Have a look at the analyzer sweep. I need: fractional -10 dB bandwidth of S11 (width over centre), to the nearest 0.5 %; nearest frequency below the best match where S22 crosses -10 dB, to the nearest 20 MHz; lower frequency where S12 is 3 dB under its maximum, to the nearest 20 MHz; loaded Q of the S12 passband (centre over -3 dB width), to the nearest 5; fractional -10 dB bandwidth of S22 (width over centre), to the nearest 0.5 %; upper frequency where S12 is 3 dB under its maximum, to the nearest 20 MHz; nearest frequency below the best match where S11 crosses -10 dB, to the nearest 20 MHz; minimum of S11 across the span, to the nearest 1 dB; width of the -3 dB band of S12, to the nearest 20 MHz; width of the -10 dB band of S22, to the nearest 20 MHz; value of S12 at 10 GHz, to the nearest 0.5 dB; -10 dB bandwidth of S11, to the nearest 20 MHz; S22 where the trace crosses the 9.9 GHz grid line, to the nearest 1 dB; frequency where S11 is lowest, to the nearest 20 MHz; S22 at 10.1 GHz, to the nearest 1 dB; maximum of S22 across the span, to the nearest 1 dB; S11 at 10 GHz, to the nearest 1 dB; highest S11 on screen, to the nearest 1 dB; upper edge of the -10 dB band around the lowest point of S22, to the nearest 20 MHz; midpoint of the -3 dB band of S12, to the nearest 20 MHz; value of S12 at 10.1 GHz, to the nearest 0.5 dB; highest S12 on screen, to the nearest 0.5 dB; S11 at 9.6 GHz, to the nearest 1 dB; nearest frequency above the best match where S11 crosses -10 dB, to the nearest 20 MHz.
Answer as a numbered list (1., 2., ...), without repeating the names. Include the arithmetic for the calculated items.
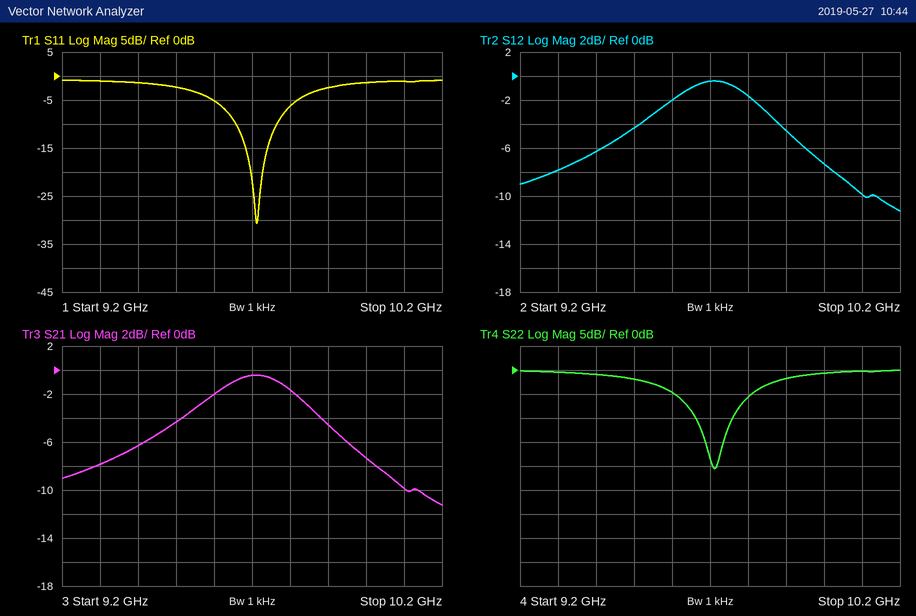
1. 100 MHz / 9.71 GHz ≈ 1.0 %
2. 9.66 GHz
3. 9.54 GHz
4. 9.7 GHz / 320 MHz ≈ 30
5. 100 MHz / 9.71 GHz ≈ 1.0 %
6. 9.86 GHz
7. 9.66 GHz
8. -31 dB
9. 9.86 GHz − 9.54 GHz = 320 MHz
10. 9.76 GHz − 9.66 GHz = 100 MHz
11. -7.5 dB
12. 9.76 GHz − 9.66 GHz = 100 MHz
13. -2 dB
14. 9.72 GHz
15. 0 dB
16. 0 dB
17. -1 dB
18. -1 dB
19. 9.76 GHz
20. 9.70 GHz
21. -10.0 dB
22. -0.5 dB
23. -5 dB
24. 9.76 GHz
